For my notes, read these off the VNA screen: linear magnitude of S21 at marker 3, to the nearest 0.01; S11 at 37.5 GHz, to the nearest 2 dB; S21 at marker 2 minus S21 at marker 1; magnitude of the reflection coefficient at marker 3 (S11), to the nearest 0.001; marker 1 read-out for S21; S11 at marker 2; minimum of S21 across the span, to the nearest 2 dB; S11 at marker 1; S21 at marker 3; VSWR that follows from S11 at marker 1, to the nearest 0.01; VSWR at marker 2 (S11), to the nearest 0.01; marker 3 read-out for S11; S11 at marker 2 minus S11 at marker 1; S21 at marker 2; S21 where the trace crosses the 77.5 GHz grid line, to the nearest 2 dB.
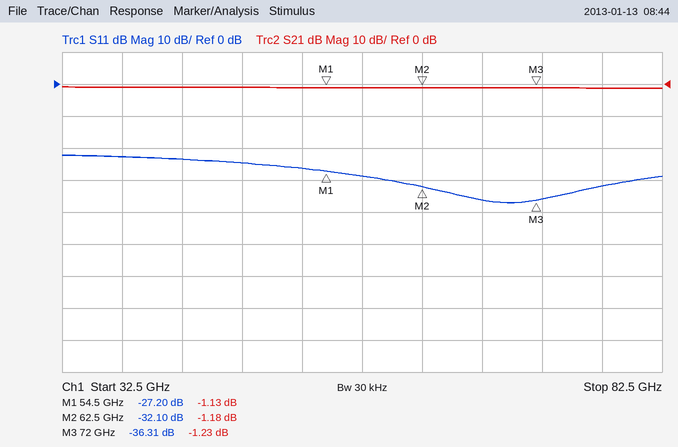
0.87
-22 dB
-0.05 dB
0.015
-1.13 dB
-32.10 dB
-2 dB
-27.20 dB
-1.23 dB
1.09
1.05
-36.31 dB
-4.90 dB
-1.18 dB
-2 dB
